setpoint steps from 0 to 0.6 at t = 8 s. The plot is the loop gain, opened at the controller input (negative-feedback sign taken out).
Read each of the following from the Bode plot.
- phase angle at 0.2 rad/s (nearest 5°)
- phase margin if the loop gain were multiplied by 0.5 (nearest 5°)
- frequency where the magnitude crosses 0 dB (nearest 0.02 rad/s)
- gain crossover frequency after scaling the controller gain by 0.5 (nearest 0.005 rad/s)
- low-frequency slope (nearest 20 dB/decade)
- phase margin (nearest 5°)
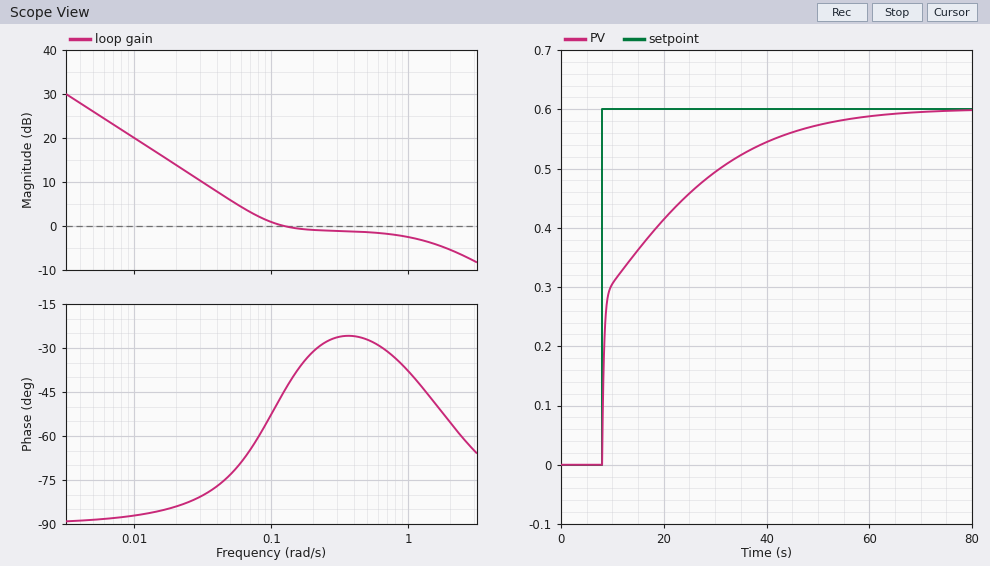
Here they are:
-30°
105°
0.12 rad/s
0.050 rad/s
-20 dB/decade
135°
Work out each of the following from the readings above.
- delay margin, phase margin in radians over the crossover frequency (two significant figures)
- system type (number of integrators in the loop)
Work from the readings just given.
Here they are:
20 s
1
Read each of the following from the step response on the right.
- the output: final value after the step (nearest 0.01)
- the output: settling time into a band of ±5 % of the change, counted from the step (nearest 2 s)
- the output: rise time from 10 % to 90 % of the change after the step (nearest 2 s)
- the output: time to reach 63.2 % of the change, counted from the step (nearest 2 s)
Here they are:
0.60
40 s
30 s
8 s
